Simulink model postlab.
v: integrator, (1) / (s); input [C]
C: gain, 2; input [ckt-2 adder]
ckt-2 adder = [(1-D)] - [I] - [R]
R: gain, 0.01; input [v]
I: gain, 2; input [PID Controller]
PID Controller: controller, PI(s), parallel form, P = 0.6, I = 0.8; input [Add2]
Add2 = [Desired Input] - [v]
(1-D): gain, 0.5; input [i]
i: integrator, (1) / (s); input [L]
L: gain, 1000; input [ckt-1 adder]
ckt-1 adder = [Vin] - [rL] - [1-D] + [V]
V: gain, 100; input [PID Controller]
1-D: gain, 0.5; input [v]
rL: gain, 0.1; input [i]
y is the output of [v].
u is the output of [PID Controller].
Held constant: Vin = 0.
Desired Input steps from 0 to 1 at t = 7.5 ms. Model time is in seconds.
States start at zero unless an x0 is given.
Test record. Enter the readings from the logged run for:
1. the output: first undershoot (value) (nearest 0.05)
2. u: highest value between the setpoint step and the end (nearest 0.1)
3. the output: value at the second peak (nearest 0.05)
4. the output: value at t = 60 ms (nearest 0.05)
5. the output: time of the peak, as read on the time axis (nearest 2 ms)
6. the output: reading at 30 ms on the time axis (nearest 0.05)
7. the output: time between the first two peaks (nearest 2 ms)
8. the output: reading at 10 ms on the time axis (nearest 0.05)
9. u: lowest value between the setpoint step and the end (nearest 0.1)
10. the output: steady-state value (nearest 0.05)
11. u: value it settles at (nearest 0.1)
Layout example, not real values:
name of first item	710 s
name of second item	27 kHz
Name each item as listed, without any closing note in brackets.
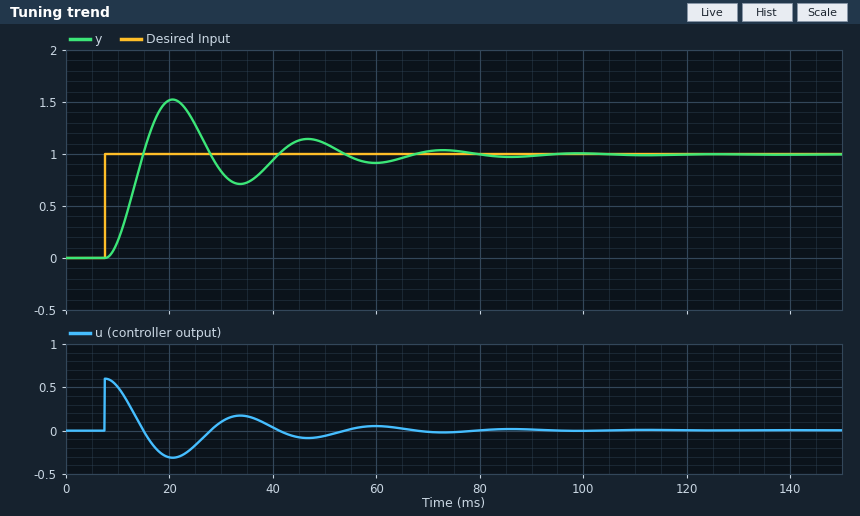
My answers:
the output: first undershoot (value)	0.70
u: highest value between the setpoint step and the end	0.6
the output: value at the second peak	1.15
the output: value at t = 60 ms	0.90
the output: time of the peak, as read on the time axis	20 ms
the output: reading at 30 ms on the time axis	0.85
the output: time between the first two peaks	26 ms
the output: reading at 10 ms on the time axis	0.15
u: lowest value between the setpoint step and the end	-0.3
the output: steady-state value	1.00
u: value it settles at	0.0
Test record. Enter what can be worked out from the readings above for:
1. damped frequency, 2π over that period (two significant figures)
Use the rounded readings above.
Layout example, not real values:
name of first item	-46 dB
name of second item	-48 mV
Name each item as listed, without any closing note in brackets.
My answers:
damped frequency, 2π over that period	0.24 rad/ms
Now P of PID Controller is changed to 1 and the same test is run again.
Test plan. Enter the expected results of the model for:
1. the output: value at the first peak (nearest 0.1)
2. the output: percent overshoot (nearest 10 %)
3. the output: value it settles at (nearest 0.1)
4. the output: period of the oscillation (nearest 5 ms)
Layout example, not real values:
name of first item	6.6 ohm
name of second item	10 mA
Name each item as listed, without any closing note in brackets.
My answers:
the output: value at the first peak	1.6
the output: percent overshoot	60 %
the output: value it settles at	1.0
the output: period of the oscillation	20 ms
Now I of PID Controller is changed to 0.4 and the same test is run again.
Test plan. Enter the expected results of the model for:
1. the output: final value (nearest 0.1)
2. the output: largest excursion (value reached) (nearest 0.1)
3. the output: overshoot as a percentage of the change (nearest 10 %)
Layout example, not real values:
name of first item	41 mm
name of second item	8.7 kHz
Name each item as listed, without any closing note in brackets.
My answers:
the output: final value	1.0
the output: largest excursion (value reached)	1.5
the output: overshoot as a percentage of the change	50 %
